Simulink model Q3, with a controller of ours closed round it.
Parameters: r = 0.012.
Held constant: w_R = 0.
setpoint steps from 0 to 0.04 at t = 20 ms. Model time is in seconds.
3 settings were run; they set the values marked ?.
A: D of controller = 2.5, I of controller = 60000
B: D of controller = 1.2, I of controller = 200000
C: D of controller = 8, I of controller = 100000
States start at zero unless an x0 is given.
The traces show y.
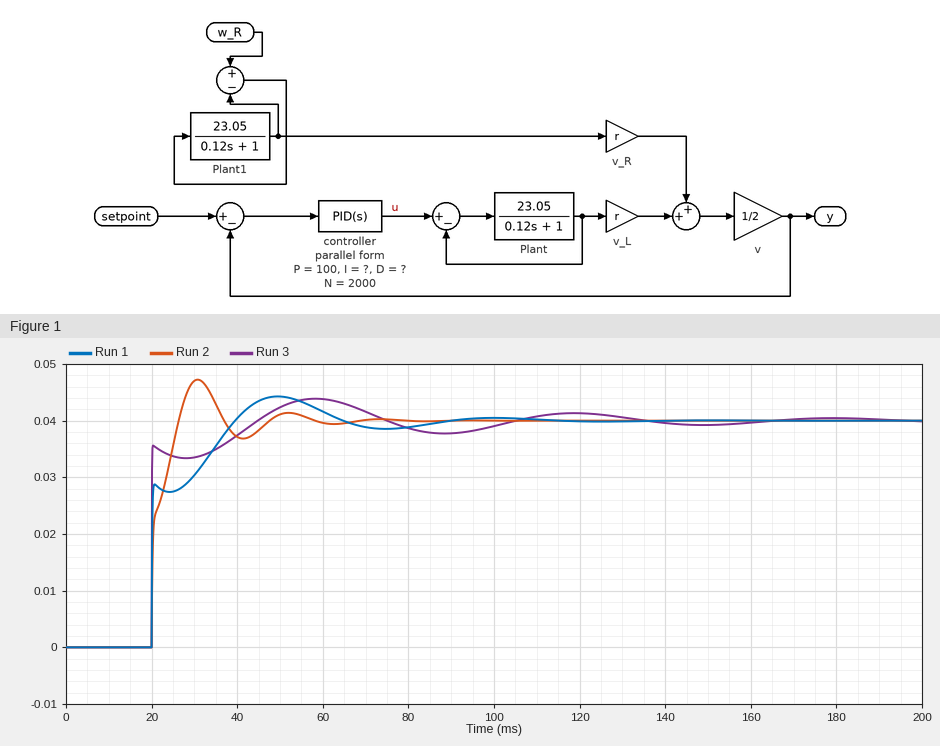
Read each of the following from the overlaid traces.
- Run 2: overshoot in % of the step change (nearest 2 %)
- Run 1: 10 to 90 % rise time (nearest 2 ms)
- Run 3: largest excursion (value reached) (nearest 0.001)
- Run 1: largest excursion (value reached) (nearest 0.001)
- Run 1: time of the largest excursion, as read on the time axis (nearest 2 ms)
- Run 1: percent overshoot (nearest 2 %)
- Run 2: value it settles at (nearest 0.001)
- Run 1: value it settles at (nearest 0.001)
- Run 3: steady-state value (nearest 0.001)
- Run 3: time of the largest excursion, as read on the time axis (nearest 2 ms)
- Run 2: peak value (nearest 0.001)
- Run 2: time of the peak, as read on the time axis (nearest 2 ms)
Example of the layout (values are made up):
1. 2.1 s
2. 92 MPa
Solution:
1. 18 %
2. 16 ms
3. 0.044
4. 0.044
5. 50 ms
6. 10 %
7. 0.040
8. 0.040
9. 0.040
10. 58 ms
11. 0.047
12. 30 ms
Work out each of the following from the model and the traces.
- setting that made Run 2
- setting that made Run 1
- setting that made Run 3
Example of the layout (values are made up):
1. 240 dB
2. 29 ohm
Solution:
1. B
2. A
3. C
